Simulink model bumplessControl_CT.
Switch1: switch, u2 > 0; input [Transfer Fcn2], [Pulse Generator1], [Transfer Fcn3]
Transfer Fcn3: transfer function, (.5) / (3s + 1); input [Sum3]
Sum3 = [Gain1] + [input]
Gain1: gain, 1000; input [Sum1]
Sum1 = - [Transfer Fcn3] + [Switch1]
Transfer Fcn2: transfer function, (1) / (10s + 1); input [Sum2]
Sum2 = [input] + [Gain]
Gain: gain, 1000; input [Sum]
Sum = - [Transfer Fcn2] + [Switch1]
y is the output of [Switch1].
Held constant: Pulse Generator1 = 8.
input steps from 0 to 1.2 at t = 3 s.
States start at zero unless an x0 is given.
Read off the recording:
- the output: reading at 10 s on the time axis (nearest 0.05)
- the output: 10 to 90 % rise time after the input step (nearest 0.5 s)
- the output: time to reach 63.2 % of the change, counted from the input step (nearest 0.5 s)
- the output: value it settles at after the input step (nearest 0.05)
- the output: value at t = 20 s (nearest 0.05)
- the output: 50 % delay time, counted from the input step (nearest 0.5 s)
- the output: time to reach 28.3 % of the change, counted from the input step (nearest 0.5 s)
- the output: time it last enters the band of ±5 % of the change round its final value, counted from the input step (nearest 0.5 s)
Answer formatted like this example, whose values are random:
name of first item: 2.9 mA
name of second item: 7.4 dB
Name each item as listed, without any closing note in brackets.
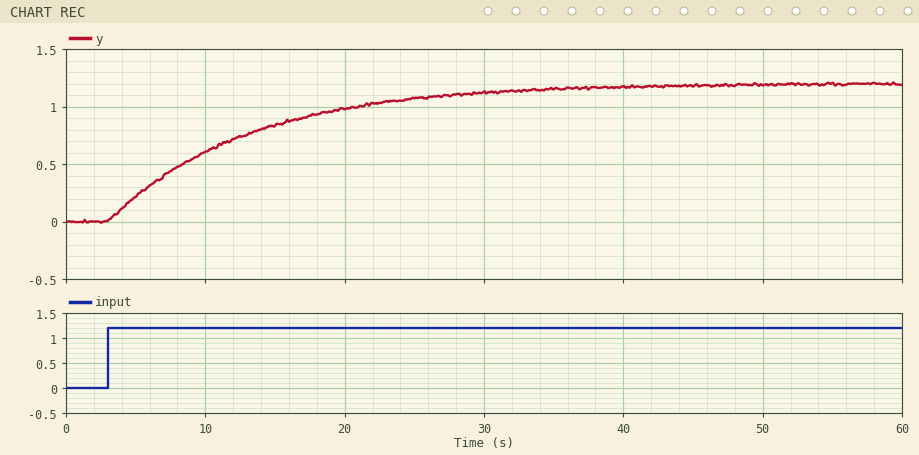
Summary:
the output: reading at 10 s on the time axis: 0.60
the output: 10 to 90 % rise time after the input step: 22.0 s
the output: time to reach 63.2 % of the change, counted from the input step: 10.0 s
the output: value it settles at after the input step: 1.20
the output: value at t = 20 s: 1.00
the output: 50 % delay time, counted from the input step: 7.0 s
the output: time to reach 28.3 % of the change, counted from the input step: 3.5 s
the output: time it last enters the band of ±5 % of the change round its final value, counted from the input step: 30.0 s
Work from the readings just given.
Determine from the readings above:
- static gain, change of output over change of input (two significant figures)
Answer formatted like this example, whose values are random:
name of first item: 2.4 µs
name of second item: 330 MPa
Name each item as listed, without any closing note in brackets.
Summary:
static gain, change of output over change of input: 1.0
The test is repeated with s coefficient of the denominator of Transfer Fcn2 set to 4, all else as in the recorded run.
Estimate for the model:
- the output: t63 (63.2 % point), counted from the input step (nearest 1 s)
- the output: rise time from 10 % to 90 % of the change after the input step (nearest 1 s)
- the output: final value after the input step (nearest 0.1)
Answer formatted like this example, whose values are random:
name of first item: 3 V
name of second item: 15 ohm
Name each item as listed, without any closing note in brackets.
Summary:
the output: t63 (63.2 % point), counted from the input step: 4 s
the output: rise time from 10 % to 90 % of the change after the input step: 9 s
the output: final value after the input step: 1.2
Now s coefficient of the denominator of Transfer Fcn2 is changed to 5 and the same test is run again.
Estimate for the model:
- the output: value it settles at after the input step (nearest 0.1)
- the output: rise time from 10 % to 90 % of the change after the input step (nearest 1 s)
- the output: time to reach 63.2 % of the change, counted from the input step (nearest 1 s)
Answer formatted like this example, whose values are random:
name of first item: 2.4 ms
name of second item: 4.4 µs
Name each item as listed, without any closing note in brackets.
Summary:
the output: value it settles at after the input step: 1.2
the output: rise time from 10 % to 90 % of the change after the input step: 11 s
the output: time to reach 63.2 % of the change, counted from the input step: 5 s
